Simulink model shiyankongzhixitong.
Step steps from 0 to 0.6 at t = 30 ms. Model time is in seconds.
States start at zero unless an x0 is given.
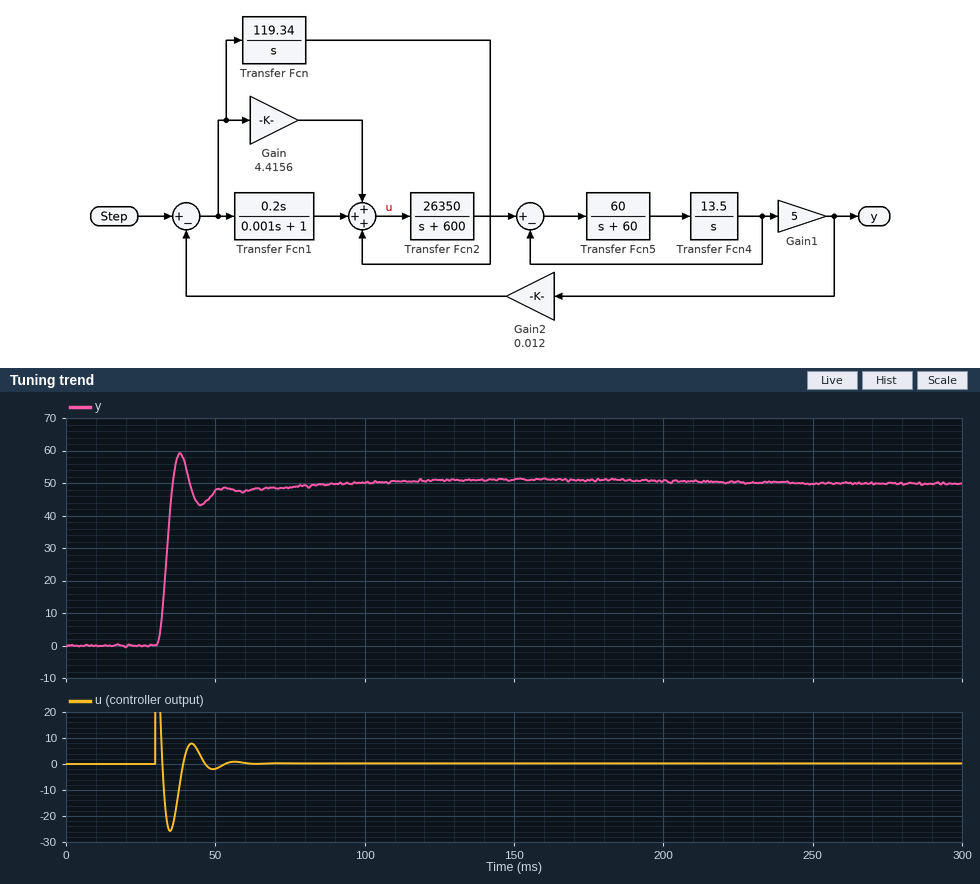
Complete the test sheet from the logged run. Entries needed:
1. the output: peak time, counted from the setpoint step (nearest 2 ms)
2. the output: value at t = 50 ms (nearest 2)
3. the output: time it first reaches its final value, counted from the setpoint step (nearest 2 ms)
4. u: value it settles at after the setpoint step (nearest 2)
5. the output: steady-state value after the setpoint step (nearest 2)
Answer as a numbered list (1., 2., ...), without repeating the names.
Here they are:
1. 8 ms
2. 48
3. 6 ms
4. 0
5. 50
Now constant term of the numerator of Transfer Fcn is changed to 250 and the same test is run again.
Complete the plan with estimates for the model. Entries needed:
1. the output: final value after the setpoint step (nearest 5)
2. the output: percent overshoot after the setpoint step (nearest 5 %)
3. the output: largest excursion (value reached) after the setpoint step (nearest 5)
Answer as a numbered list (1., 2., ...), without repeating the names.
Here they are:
1. 50
2. 20 %
3. 60
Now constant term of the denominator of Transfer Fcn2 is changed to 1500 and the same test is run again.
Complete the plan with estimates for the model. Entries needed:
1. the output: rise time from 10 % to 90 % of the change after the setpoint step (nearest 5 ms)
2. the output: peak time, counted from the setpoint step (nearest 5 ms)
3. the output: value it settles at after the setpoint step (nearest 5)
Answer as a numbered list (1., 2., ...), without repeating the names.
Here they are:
1. 35 ms
2. 135 ms
3. 50
